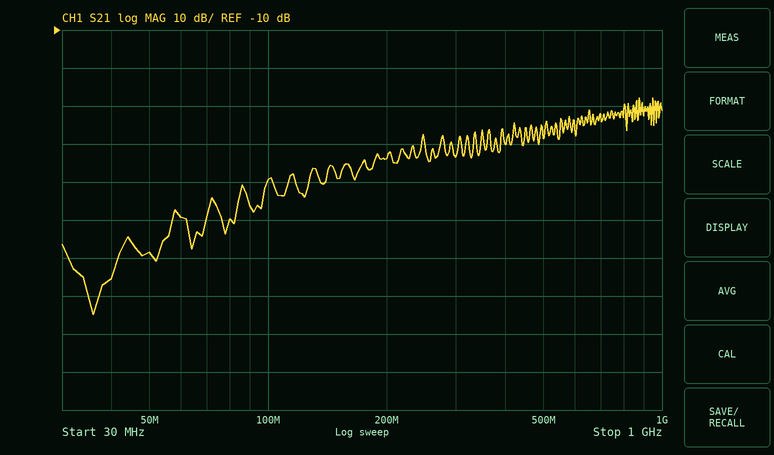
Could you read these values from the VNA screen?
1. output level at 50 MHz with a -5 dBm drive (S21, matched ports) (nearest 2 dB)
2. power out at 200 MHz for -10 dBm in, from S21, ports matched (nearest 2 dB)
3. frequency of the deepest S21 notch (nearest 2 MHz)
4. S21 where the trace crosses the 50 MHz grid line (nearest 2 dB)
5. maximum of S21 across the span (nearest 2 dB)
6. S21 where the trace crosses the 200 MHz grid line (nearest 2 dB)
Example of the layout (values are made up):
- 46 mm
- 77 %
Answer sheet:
- -74 dBm
- -54 dBm
- 36 MHz
- -68 dB
- -28 dB
- -44 dB
